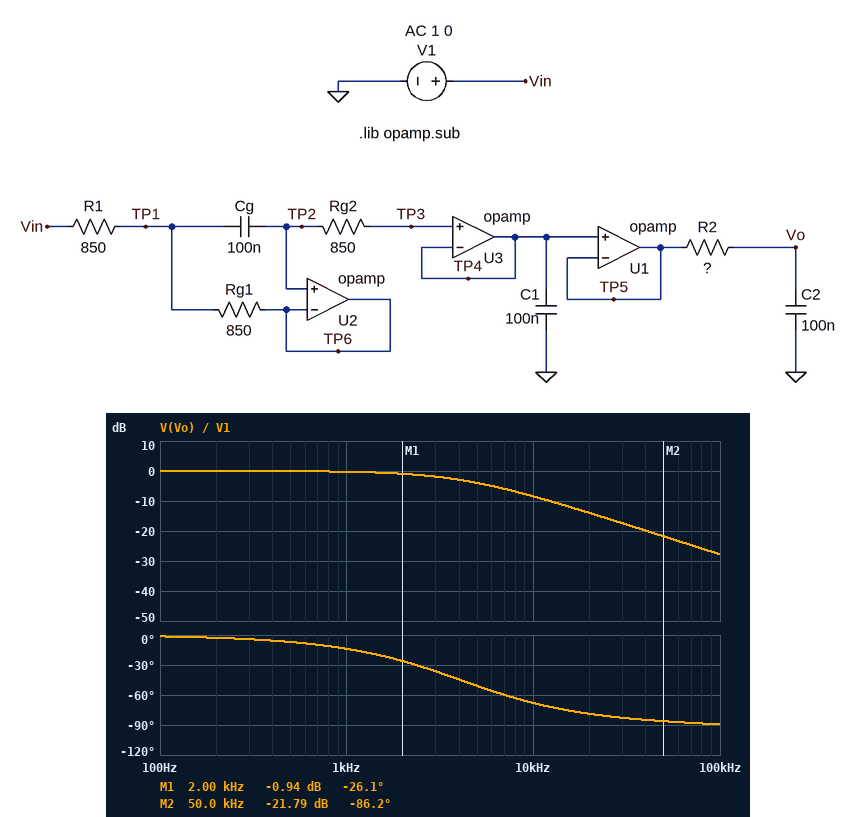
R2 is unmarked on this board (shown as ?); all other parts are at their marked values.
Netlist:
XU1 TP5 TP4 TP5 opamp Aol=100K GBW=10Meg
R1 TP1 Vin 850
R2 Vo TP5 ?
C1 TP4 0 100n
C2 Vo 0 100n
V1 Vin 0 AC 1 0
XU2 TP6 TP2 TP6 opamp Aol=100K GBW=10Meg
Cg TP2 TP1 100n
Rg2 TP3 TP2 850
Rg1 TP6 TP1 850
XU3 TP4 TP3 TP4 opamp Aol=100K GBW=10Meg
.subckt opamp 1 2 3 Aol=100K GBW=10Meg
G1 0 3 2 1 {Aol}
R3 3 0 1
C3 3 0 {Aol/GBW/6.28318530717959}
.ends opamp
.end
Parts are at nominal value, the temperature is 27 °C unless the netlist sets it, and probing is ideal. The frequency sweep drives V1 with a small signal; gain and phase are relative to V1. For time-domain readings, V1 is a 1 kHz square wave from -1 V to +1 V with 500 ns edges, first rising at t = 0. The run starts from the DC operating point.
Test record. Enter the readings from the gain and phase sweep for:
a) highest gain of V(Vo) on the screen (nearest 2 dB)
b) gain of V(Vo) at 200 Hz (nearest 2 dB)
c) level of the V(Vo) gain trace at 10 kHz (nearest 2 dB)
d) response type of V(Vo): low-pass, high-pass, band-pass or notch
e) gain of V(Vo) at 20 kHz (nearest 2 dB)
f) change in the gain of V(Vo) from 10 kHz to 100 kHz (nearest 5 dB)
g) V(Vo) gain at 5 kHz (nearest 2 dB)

0 dB
0 dB
-8 dB
low-pass
-14 dB
-20 dB
-4 dB
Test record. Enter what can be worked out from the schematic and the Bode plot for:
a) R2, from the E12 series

390 Ω
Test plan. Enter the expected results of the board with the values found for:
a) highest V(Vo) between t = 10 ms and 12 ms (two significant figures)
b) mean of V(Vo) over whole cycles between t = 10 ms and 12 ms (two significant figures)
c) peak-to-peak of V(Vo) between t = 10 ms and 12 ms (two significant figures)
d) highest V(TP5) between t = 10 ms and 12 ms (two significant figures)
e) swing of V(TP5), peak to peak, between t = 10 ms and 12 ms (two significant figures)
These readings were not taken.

2.0 V
1.0 V
2.0 V
2.0 V
2.0 V
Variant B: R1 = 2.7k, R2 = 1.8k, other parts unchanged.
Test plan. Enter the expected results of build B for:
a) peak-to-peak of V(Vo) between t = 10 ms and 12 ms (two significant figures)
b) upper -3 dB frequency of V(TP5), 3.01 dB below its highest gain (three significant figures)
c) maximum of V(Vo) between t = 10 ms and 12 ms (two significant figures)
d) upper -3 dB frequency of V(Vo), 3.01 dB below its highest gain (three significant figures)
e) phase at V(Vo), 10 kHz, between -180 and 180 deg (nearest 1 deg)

1.8 V
2.27 MHz
1.9 V
884 Hz
-85 deg
